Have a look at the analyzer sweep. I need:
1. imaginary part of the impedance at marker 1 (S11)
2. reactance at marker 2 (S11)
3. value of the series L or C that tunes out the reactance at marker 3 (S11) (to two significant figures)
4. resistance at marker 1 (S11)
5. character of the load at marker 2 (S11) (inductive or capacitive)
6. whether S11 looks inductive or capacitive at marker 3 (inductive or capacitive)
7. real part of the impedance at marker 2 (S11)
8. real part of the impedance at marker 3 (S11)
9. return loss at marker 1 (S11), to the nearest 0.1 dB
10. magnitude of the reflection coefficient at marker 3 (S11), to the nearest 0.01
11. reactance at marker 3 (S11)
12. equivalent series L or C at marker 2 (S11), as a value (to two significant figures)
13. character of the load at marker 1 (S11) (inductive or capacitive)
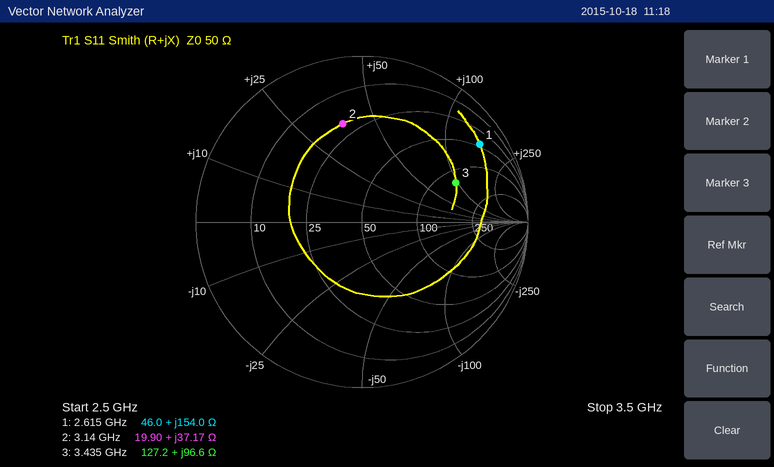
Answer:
+154.0 Ω
+37.17 Ω
480 fF
46.0 Ω
inductive
inductive
19.90 Ω
127.2 Ω
1.4 dB
0.61
+96.6 Ω
1.9 nH
inductive
